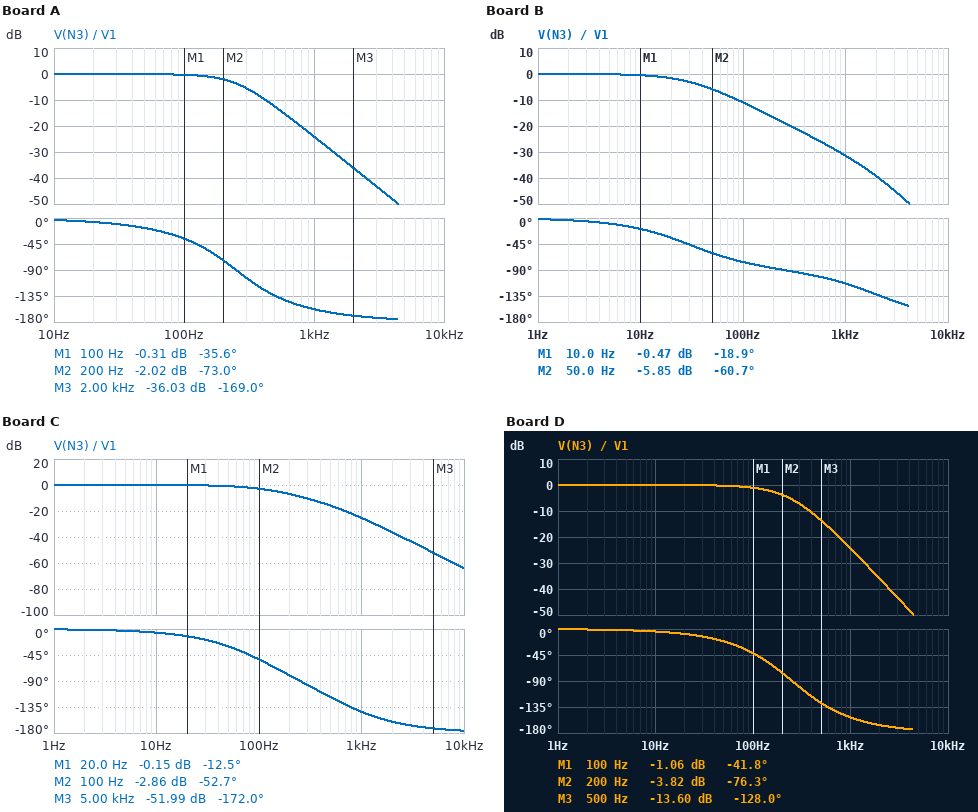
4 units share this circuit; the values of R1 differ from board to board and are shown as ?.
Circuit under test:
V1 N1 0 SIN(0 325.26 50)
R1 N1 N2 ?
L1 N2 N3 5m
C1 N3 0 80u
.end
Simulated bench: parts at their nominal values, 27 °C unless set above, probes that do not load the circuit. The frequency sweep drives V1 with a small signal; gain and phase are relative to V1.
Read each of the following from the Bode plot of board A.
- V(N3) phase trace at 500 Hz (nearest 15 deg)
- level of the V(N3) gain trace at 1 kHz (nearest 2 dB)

-135 deg
-24 dB
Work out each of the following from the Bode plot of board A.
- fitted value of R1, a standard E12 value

12 Ω
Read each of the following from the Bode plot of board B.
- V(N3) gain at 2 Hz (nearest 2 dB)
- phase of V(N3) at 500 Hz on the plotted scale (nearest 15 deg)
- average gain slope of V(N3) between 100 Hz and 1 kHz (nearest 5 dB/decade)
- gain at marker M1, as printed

0 dB
-105 deg
-20 dB/decade
-0.47 dB
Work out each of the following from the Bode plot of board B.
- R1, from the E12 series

68 Ω
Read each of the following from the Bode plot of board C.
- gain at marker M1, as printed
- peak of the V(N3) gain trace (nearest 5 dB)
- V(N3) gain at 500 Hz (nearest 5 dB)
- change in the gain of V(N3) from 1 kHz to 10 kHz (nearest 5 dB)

-0.15 dB
0 dB
-15 dB
-40 dB
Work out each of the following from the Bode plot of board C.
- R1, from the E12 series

22 Ω
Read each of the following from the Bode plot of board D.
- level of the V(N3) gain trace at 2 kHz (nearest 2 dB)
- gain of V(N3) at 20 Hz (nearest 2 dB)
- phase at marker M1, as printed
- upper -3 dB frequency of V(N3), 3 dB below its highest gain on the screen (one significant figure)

-36 dB
0 dB
-41.8 deg
200 Hz
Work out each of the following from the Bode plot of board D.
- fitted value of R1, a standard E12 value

15 Ω
